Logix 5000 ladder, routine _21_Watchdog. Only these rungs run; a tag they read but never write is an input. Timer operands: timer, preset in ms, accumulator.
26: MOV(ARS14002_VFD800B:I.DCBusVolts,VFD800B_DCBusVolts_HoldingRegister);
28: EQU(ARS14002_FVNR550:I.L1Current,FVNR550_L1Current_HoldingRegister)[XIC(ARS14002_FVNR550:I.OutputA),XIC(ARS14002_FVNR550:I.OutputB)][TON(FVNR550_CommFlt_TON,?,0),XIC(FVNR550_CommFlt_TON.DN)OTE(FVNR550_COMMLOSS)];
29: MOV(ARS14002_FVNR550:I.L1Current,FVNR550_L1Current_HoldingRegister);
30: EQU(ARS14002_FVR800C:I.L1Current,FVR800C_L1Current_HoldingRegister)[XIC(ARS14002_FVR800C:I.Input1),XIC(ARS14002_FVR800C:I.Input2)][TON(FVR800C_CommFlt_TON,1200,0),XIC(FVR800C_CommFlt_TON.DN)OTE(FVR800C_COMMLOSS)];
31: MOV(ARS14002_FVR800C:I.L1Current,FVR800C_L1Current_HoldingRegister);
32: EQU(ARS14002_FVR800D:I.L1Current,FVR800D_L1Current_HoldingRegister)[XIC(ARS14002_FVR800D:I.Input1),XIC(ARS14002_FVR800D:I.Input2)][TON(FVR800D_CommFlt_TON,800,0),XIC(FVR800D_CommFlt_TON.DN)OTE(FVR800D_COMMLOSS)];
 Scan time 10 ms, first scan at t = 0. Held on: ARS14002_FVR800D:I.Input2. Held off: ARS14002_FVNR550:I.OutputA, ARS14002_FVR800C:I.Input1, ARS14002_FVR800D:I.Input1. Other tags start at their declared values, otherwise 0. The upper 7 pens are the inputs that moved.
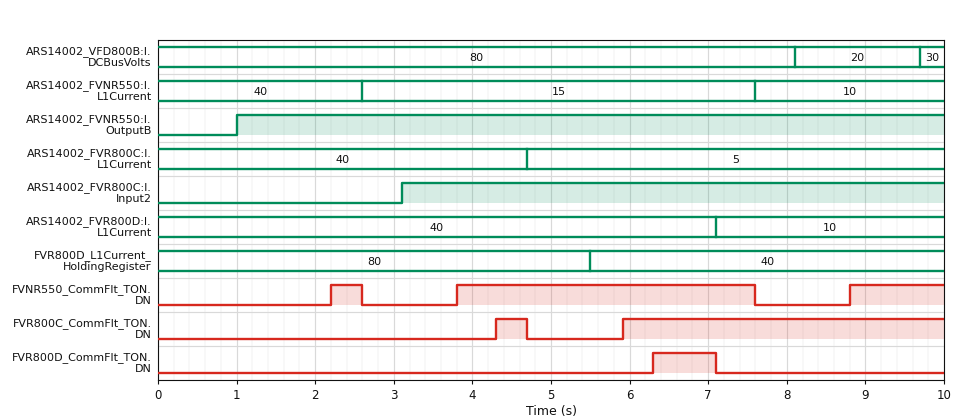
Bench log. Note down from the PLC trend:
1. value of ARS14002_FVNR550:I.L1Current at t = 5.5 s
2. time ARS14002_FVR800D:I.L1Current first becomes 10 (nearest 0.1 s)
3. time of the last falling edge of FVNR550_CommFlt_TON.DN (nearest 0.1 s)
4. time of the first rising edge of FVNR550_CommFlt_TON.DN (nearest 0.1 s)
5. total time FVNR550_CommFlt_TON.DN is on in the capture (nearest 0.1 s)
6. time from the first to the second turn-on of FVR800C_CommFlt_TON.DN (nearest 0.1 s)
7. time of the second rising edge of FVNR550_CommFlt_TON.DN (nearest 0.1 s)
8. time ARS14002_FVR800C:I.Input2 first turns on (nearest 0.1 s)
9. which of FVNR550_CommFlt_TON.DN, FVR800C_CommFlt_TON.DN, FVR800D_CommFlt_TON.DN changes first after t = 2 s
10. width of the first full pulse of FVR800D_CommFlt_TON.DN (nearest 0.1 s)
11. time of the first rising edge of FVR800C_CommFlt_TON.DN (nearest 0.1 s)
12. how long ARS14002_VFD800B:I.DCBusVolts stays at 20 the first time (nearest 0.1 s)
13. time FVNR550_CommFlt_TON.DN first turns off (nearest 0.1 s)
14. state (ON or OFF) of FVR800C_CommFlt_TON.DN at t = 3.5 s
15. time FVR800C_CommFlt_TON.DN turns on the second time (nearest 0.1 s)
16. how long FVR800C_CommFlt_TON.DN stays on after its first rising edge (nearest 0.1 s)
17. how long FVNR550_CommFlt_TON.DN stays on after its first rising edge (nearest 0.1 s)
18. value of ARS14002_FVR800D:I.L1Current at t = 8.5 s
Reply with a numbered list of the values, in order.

1. 15
2. 7.1 s
3. 7.6 s
4. 2.2 s
5. 5.4 s
6. 1.6 s
7. 3.8 s
8. 3.1 s
9. FVNR550_CommFlt_TON.DN
10. 0.8 s
11. 4.3 s
12. 1.6 s
13. 2.6 s
14. OFF
15. 5.9 s
16. 0.4 s
17. 0.4 s
18. 10
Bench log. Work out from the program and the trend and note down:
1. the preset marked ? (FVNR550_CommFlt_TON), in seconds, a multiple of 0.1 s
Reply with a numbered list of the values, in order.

1. 1.2 s
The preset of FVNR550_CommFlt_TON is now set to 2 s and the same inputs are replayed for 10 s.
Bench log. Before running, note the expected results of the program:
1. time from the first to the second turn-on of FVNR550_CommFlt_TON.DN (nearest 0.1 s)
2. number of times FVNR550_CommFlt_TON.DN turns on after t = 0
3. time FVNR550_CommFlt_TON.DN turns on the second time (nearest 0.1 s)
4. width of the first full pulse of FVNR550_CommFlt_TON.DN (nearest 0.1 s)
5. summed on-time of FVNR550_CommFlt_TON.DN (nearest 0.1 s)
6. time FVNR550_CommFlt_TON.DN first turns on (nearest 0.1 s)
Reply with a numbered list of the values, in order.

1. 5.0 s
2. 2
3. 9.6 s
4. 3.0 s
5. 3.4 s
6. 4.6 s
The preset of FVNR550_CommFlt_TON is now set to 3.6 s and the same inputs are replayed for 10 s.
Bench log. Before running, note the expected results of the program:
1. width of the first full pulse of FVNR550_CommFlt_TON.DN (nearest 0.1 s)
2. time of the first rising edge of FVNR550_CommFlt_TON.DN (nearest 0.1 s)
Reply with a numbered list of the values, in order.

1. 1.4 s
2. 6.2 s
